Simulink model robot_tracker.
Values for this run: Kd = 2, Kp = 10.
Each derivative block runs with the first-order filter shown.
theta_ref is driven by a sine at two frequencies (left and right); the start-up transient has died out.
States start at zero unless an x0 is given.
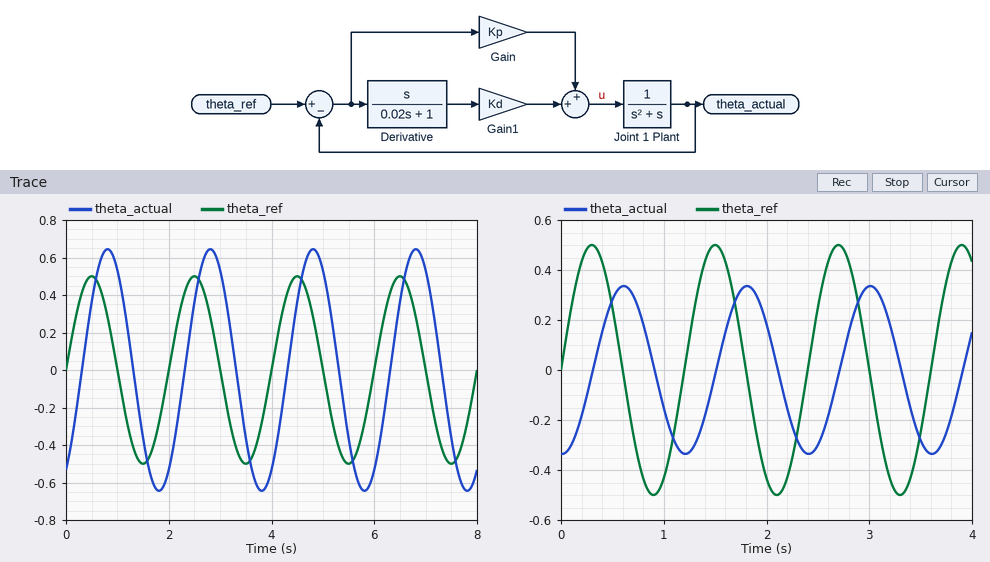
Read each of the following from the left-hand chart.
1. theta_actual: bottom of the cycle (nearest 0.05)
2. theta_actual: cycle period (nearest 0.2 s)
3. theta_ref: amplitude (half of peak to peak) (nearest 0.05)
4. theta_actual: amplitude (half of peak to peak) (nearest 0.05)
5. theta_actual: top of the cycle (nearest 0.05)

-0.65
2.0 s
0.50
0.65
0.65
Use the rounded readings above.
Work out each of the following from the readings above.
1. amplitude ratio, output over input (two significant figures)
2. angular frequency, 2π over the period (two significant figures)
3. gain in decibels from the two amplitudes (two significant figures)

1.3
3.1 rad/s
2.3 dB
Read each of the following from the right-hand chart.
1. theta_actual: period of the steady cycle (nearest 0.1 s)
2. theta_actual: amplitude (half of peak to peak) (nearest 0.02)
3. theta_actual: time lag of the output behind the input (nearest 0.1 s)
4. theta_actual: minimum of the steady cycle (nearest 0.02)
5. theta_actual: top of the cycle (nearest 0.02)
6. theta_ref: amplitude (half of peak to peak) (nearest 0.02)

1.2 s
0.34
0.3 s
-0.34
0.34
0.50
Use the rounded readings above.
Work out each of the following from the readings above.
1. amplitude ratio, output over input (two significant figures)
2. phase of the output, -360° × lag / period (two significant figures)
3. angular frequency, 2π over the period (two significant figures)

0.68
-90°
5.2 rad/s
